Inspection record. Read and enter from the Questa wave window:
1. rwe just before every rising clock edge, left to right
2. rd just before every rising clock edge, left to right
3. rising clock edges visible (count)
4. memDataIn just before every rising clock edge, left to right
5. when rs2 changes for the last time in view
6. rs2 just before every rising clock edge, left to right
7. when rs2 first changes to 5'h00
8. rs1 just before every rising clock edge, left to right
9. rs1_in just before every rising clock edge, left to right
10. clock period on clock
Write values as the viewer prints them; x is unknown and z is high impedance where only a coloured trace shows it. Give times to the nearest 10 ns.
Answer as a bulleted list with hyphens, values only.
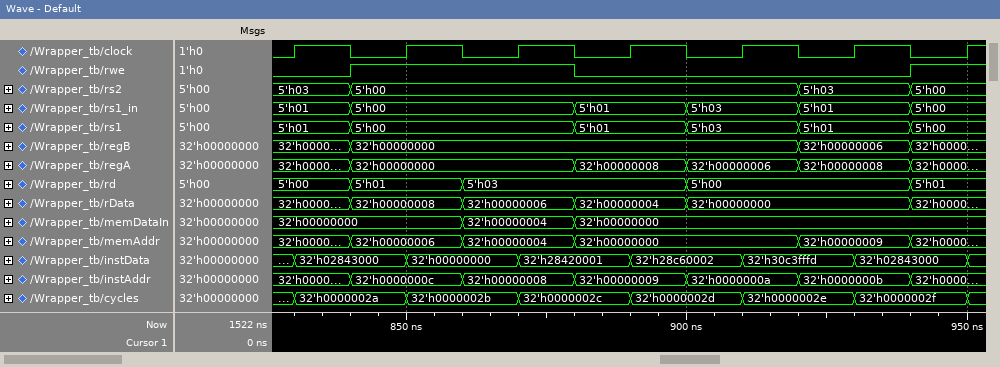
- 0 1 1 0 0 0 1
- 5'h00, 5'h01, 5'h03, 5'h03, 5'h00, 5'h00, 5'h01
- 7
- 32'h00000000, 32'h00000000, 32'h00000004, 32'h00000000, 32'h00000000, 32'h00000000, 32'h00000000
- 940 ns
- 5'h03, 5'h00, 5'h00, 5'h00, 5'h00, 5'h03, 5'h00
- 840 ns
- 5'h01, 5'h00, 5'h00, 5'h01, 5'h03, 5'h01, 5'h00
- 5'h01, 5'h00, 5'h00, 5'h01, 5'h03, 5'h01, 5'h00
- 20 ns
